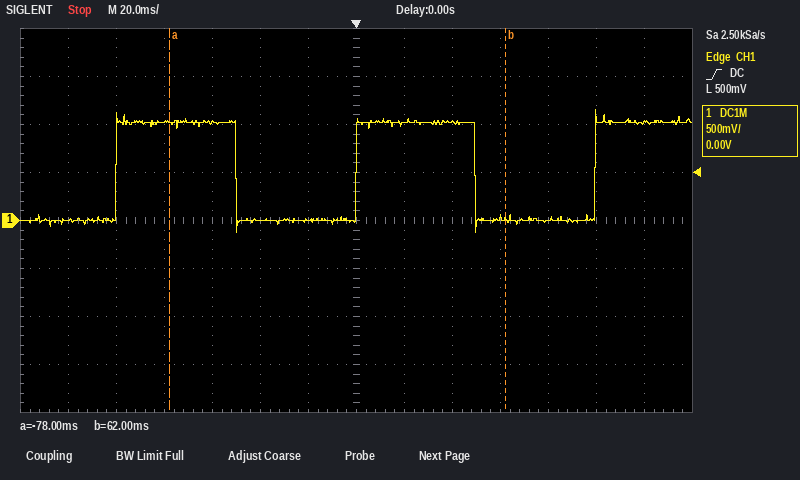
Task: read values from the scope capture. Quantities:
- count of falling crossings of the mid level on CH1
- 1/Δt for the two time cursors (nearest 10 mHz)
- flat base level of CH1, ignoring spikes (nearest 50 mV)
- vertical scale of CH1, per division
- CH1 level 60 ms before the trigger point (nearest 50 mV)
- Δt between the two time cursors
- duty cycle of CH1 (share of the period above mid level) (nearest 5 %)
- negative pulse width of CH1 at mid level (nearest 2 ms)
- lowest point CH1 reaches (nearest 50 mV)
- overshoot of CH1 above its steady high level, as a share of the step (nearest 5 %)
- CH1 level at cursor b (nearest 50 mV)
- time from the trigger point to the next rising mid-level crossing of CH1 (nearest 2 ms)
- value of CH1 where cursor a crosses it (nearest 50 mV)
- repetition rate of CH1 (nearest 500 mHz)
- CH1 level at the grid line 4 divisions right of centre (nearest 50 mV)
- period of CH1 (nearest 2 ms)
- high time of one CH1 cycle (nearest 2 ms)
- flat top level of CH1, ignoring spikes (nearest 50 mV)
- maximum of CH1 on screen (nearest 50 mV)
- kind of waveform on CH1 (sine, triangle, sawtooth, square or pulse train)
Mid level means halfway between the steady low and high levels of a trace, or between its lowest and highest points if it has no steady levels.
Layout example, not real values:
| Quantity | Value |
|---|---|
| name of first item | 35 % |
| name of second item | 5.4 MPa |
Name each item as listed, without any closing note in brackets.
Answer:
| Quantity | Value |
|---|---|
| count of falling crossings of the mid level on CH1 | 2 |
| 1/Δt for the two time cursors | 7.14 Hz |
| flat base level of CH1, ignoring spikes | 0 mV |
| vertical scale of CH1, per division | 500 mV |
| CH1 level 60 ms before the trigger point | 1.00 V |
| Δt between the two time cursors | 140 ms |
| duty cycle of CH1 (share of the period above mid level) | 50 % |
| negative pulse width of CH1 at mid level | 50 ms |
| lowest point CH1 reaches | -100 mV |
| overshoot of CH1 above its steady high level, as a share of the step | 15 % |
| CH1 level at cursor b | 0 mV |
| time from the trigger point to the next rising mid-level crossing of CH1 | 100 ms |
| value of CH1 where cursor a crosses it | 1.00 V |
| repetition rate of CH1 | 10.0 Hz |
| CH1 level at the grid line 4 divisions right of centre | 0 mV |
| period of CH1 | 100 ms |
| high time of one CH1 cycle | 50 ms |
| flat top level of CH1, ignoring spikes | 1.00 V |
| maximum of CH1 on screen | 1.15 V |
| kind of waveform on CH1 | square |
